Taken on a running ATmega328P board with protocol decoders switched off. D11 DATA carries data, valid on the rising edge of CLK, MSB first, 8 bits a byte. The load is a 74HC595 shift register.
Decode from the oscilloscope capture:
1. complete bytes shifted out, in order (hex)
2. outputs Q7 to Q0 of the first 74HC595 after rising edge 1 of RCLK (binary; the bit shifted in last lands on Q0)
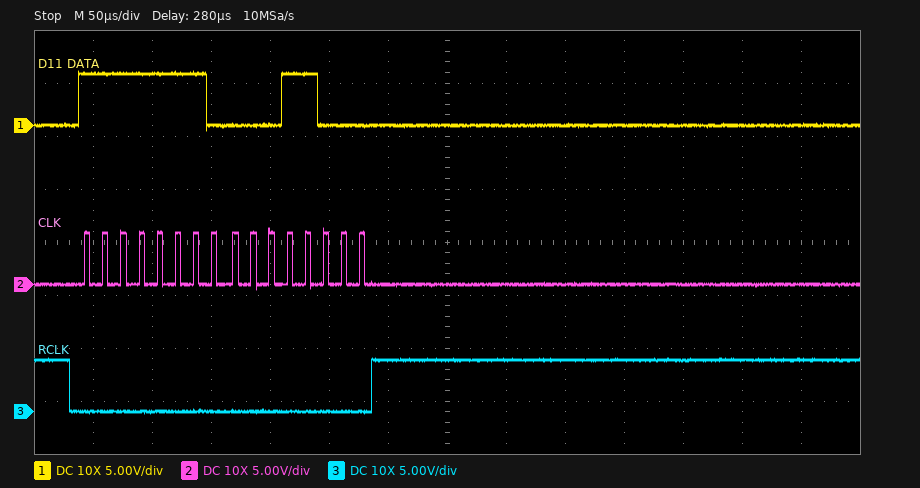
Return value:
FE 18
00011000
